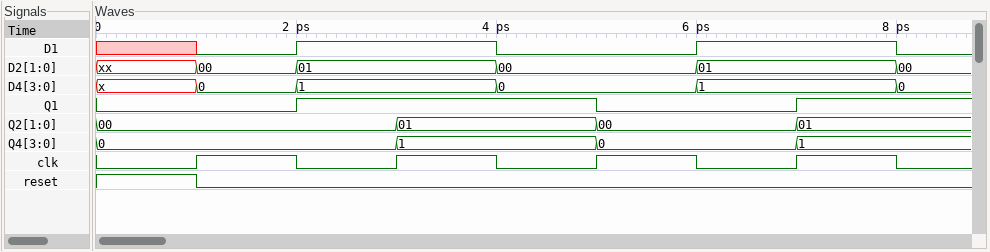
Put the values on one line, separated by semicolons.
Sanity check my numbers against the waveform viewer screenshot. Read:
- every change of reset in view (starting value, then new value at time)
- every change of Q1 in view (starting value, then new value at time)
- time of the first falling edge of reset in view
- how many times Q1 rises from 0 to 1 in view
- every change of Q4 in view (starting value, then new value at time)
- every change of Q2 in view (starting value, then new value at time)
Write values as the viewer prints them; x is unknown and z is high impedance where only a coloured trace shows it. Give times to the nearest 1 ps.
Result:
1, 0 at 1 ps; 0, 1 at 2 ps, 0 at 5 ps, 1 at 7 ps; 1 ps; 2; 0, 1 at 3 ps, 0 at 5 ps, 1 at 7 ps; 00, 01 at 3 ps, 00 at 5 ps, 01 at 7 ps
